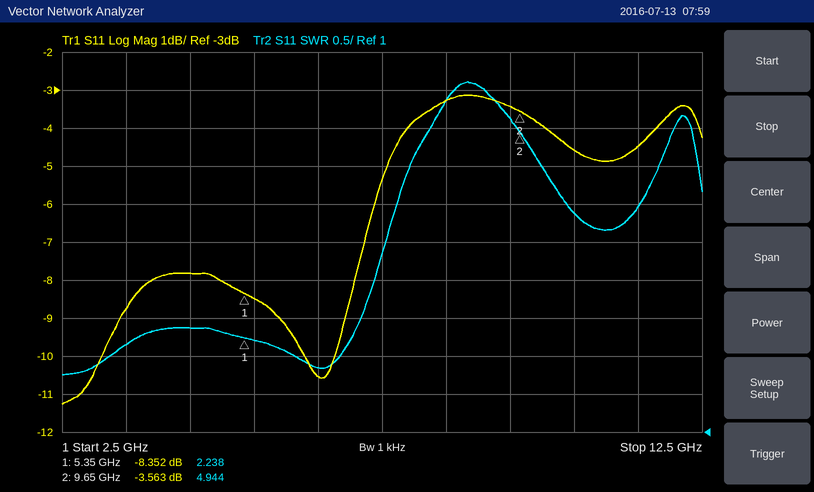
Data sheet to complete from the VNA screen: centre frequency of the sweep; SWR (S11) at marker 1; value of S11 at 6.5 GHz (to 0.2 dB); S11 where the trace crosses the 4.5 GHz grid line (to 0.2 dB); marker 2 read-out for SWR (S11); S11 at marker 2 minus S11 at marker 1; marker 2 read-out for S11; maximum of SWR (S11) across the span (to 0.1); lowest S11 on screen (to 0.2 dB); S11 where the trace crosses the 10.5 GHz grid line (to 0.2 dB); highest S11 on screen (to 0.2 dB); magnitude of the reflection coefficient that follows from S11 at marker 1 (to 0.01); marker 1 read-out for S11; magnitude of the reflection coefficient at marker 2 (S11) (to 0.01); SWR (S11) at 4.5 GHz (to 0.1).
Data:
7.5 GHz
2.238
-10.6 dB
-7.8 dB
4.944
4.789 dB
-3.563 dB
5.6
-11.2 dB
-4.6 dB
-3.2 dB
0.38
-8.352 dB
0.66
2.4
